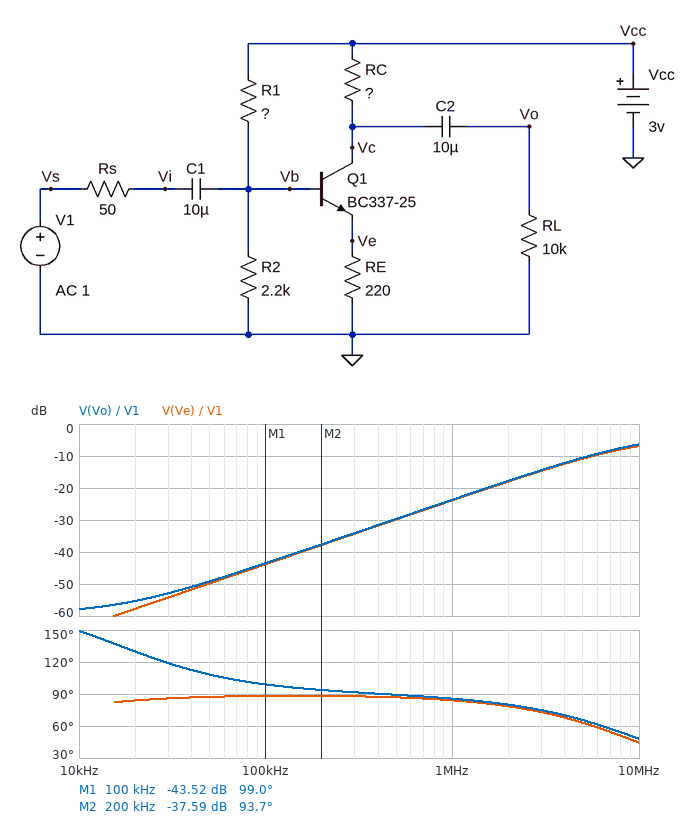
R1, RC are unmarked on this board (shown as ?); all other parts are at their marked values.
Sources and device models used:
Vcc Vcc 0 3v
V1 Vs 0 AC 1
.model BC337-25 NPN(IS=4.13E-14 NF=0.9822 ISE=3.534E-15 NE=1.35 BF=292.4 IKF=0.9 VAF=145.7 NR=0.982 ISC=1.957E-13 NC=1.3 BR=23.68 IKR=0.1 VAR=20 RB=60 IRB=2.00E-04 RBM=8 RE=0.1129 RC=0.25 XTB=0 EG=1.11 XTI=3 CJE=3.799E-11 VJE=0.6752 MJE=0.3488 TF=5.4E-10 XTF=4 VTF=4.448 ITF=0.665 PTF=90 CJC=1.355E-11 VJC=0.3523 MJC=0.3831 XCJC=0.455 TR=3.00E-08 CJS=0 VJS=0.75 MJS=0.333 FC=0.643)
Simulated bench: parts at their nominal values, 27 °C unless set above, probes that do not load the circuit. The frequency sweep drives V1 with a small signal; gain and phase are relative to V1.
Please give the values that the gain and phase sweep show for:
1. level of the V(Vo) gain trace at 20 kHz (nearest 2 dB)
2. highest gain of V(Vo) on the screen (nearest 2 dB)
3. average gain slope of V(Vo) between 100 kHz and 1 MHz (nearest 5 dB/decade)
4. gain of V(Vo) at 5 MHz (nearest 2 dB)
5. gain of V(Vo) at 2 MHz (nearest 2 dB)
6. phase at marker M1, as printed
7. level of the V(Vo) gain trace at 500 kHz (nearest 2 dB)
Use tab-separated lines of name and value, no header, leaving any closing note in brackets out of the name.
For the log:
level of the V(Vo) gain trace at 20 kHz	-56 dB
highest gain of V(Vo) on the screen	-6 dB
average gain slope of V(Vo) between 100 kHz and 1 MHz	20 dB/decade
gain of V(Vo) at 5 MHz	-10 dB
gain of V(Vo) at 2 MHz	-18 dB
phase at marker M1, as printed	99.0 deg
level of the V(Vo) gain trace at 500 kHz	-30 dB
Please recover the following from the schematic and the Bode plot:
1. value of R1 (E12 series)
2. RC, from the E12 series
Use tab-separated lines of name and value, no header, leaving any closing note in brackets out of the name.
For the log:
value of R1	18 kΩ
RC, from the E12 series	2.2 kΩ
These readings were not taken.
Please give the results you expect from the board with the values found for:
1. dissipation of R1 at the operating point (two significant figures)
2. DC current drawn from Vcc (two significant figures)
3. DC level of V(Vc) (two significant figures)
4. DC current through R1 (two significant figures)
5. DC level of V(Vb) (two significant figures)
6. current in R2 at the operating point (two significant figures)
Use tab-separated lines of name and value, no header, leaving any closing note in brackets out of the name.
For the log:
dissipation of R1 at the operating point	400 µW
DC current drawn from Vcc	150 µA
DC level of V(Vc)	3.0 V
DC current through R1	150 µA
DC level of V(Vb)	330 mV
current in R2 at the operating point	150 µA
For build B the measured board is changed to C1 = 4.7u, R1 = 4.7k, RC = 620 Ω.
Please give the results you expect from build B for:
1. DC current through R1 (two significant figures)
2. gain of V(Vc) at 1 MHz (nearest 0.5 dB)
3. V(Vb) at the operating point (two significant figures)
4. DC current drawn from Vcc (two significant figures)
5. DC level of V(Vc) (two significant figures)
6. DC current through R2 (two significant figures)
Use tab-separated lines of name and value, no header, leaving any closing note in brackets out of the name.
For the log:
DC current through R1	440 µA
gain of V(Vc) at 1 MHz	7.5 dB
V(Vb) at the operating point	950 mV
DC current drawn from Vcc	1.9 mA
DC level of V(Vc)	2.1 V
DC current through R2	430 µA
